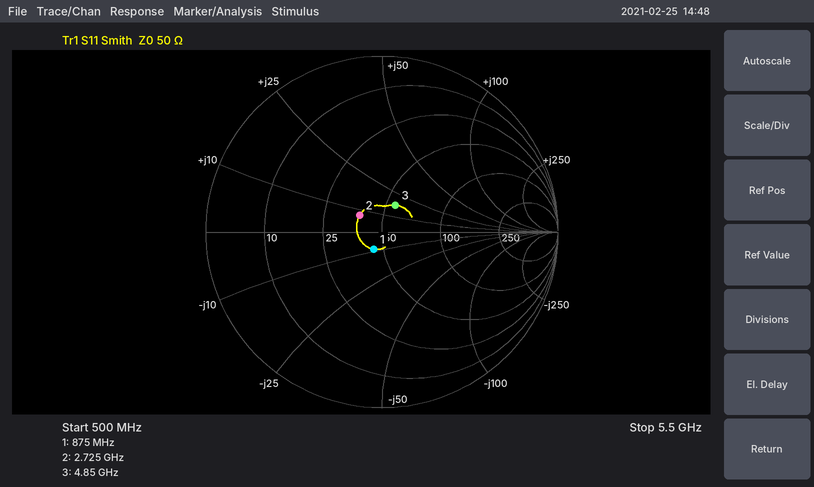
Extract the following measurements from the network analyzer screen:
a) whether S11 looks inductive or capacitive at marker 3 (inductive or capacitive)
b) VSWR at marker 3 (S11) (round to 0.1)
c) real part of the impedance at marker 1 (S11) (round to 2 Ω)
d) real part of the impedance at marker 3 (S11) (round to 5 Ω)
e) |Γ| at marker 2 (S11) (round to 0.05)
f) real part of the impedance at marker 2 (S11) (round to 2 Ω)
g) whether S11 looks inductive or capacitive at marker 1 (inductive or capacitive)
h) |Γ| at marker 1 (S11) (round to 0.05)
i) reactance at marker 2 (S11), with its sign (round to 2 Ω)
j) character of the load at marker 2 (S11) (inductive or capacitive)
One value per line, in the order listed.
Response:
inductive
1.4
44 Ω
55 Ω
0.15
38 Ω
capacitive
0.10
+8 Ω
inductive
